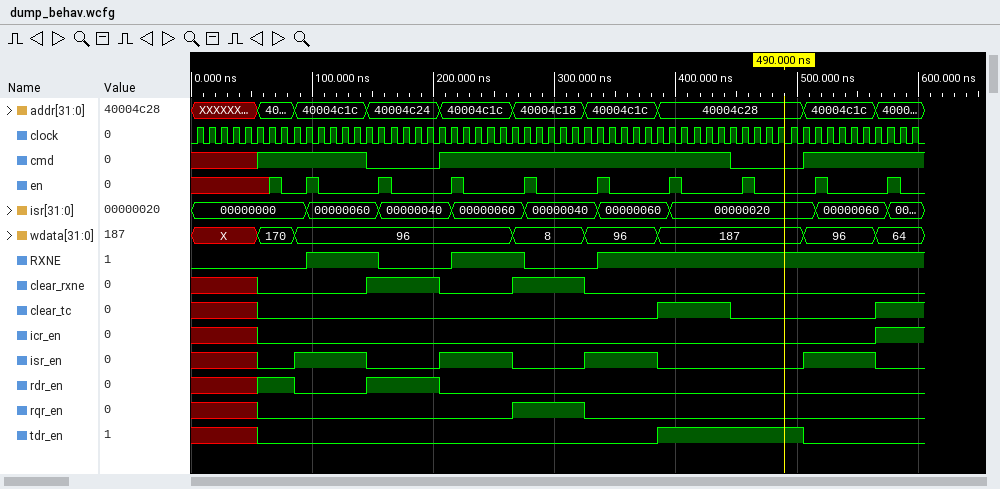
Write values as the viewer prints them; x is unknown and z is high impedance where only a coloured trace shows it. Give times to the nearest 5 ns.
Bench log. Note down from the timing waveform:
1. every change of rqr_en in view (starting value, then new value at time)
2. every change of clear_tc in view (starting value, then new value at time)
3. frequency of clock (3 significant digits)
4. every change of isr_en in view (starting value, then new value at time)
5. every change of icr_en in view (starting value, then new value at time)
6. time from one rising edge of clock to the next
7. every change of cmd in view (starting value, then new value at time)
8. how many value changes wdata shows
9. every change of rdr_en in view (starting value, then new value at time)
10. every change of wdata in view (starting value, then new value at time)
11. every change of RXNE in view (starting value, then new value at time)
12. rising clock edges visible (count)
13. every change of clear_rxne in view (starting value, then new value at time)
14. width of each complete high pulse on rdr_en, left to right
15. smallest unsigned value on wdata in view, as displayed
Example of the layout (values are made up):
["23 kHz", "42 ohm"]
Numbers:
["x, 0 at 55 ns, 1 at 265 ns, 0 at 325 ns", "x, 0 at 55 ns, 1 at 385 ns, 0 at 445 ns, 1 at 565 ns", "100 MHz", "x, 0 at 55 ns, 1 at 85 ns, 0 at 145 ns, 1 at 205 ns, 0 at 265 ns, 1 at 325 ns, 0 at 385 ns, 1 at 505 ns, 0 at 565 ns", "x, 0 at 55 ns, 1 at 565 ns", "10 ns", "x, 1 at 55 ns, 0 at 145 ns, 1 at 205 ns, 0 at 445 ns, 1 at 505 ns", "7", "x, 1 at 55 ns, 0 at 85 ns, 1 at 145 ns, 0 at 205 ns", "X, 170 at 55 ns, 96 at 85 ns, 8 at 265 ns, 96 at 325 ns, 187 at 385 ns, 96 at 505 ns, 64 at 565 ns", "0, 1 at 95 ns, 0 at 155 ns, 1 at 215 ns, 0 at 275 ns, 1 at 335 ns", "60", "x, 0 at 55 ns, 1 at 145 ns, 0 at 205 ns, 1 at 265 ns, 0 at 325 ns", "60 ns", "8"]
